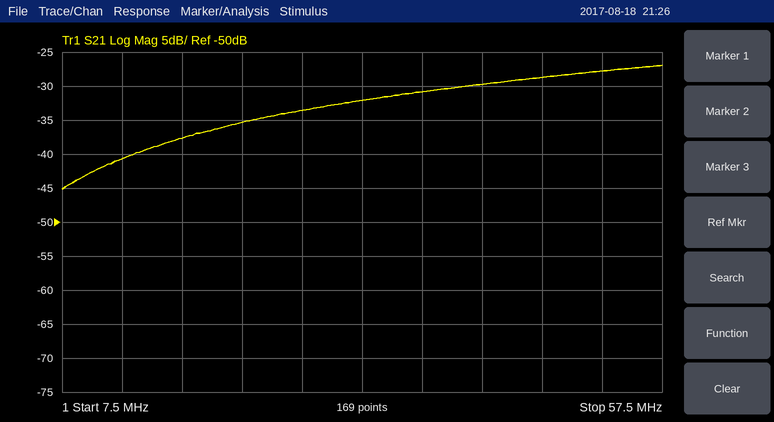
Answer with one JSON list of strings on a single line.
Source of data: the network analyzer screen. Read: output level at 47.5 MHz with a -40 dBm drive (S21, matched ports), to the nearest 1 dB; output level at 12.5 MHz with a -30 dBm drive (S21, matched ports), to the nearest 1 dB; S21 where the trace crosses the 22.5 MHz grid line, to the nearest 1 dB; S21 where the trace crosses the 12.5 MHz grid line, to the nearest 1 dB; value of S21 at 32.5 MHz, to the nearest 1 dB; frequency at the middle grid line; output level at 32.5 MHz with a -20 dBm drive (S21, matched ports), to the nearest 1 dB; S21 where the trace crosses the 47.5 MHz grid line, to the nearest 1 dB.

["-69 dBm", "-71 dBm", "-35 dB", "-41 dB", "-32 dB", "32.5 MHz", "-52 dBm", "-29 dB"]
